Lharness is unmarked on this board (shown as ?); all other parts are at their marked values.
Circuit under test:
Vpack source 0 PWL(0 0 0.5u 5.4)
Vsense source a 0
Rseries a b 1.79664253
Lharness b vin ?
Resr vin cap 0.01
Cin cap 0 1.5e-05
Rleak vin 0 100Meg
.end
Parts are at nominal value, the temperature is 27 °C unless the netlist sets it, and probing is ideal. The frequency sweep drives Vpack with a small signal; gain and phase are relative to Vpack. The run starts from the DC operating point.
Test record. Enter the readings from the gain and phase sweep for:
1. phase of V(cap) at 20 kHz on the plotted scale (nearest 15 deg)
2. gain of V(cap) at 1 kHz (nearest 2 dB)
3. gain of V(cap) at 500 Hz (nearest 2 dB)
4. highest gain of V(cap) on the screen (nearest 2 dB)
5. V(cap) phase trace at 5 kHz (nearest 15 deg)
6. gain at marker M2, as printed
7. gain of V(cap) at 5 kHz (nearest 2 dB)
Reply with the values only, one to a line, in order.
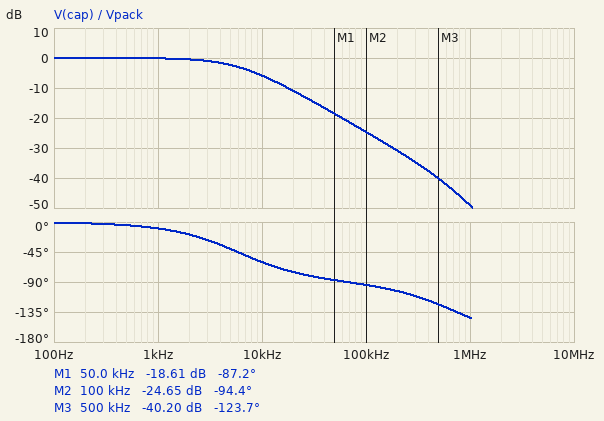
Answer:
-75 deg
0 dB
0 dB
0 dB
-45 deg
-24.65 dB
-2 dB
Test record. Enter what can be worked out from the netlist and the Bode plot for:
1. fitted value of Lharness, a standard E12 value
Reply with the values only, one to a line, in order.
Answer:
390 nH
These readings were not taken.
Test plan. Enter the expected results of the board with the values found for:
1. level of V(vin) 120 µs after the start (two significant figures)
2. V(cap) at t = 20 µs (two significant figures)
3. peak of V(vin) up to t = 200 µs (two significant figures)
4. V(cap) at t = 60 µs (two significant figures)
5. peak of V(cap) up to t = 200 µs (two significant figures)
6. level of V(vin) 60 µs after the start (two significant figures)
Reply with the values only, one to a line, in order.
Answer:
5.3 V
2.8 V
5.4 V
4.8 V
5.4 V
4.8 V
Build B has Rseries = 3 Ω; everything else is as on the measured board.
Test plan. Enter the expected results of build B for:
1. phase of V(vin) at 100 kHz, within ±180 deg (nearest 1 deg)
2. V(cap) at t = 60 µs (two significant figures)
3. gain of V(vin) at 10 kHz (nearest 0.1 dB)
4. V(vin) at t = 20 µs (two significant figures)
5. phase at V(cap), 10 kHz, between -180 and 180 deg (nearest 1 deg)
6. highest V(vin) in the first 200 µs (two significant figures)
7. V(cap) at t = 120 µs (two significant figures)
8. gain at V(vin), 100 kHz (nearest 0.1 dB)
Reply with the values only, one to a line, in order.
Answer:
-87 deg
4.0 V
-9.5 dB
1.9 V
-71 deg
5.3 V
5.0 V
-29.0 dB
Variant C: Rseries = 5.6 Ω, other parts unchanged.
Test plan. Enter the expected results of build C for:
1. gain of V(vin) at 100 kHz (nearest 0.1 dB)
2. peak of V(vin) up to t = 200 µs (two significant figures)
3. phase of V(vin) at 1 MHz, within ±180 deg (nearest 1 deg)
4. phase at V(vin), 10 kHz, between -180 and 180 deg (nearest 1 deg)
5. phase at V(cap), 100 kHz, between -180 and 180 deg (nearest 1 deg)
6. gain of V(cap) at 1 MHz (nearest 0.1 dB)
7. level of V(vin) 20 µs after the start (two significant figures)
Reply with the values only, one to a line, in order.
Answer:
-34.4 dB
4.9 V
-70 deg
-79 deg
-91 deg
-55.2 dB
1.1 V
